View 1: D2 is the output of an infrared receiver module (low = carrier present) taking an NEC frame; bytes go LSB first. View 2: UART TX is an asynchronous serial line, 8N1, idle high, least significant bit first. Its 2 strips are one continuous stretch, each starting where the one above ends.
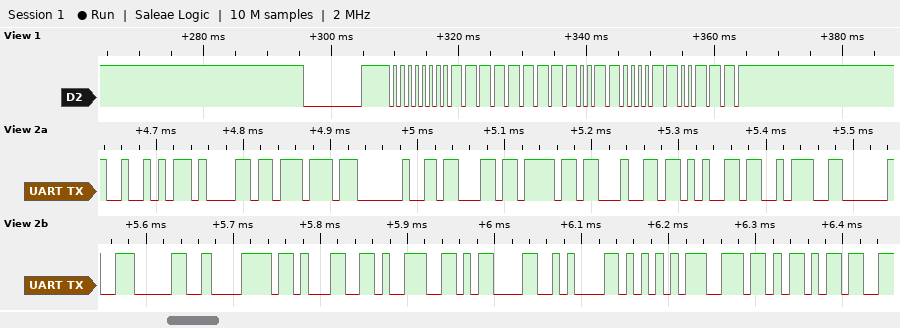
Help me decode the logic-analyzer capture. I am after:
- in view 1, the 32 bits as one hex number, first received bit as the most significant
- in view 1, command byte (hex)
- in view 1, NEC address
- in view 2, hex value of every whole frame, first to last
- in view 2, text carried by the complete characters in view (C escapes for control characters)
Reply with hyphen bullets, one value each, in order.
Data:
- 0x00FF9867
- 0x19
- 0x00
- 0x52 0x61 0x77 0x20 0x63 0x6F 0x64 0x65 0x3A 0x20 0x30 0x78 0x31 0x39 0x0D 0x0A 0x55 0x6E 0x6B
- "Raw code: 0x19\r\nUnk"
